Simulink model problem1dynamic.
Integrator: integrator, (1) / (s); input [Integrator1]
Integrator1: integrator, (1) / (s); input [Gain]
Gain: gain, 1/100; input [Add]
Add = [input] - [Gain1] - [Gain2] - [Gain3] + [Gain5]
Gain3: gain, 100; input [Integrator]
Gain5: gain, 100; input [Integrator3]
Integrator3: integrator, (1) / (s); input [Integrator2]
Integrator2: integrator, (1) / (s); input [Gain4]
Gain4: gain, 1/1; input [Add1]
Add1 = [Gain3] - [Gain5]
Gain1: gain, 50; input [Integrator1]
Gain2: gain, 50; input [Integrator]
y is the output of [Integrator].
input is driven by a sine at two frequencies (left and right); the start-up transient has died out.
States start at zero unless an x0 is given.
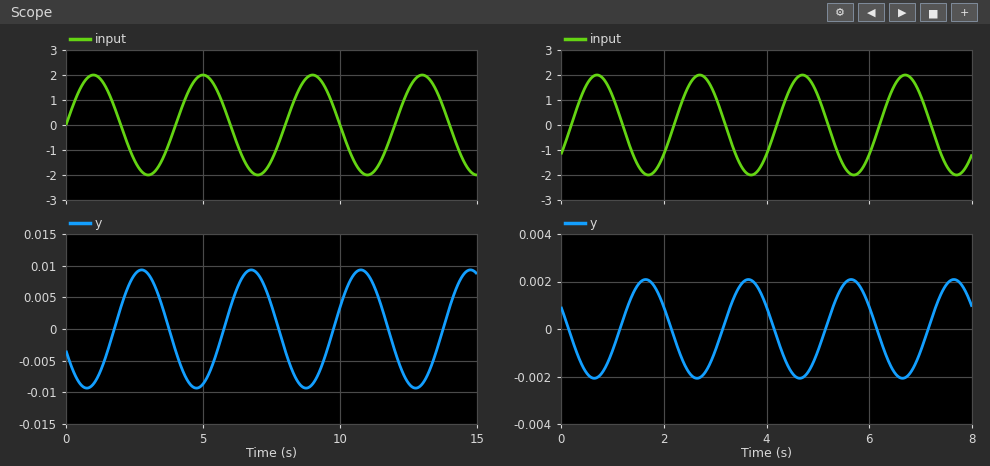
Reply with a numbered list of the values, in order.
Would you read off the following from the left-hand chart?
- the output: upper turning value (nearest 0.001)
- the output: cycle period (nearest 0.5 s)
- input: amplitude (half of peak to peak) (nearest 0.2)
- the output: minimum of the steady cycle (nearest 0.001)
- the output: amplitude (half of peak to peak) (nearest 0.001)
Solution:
1. 0.009
2. 4.0 s
3. 2.0
4. -0.009
5. 0.009
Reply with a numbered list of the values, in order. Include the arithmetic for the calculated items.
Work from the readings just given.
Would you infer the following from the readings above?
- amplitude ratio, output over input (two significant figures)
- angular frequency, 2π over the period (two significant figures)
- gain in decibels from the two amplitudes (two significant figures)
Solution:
1. 0.009 / 2 = 0.0045
2. 2π / 4 = 1.6 rad/s
3. 20 log10(0.009 / 2) = -47 dB
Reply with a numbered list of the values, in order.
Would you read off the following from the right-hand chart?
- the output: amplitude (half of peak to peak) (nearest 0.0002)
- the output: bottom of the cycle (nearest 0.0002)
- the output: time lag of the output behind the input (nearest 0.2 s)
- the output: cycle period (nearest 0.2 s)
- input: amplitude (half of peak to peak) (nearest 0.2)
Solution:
1. 0.0020
2. -0.0020
3. 1.0 s
4. 2.0 s
5. 2.0
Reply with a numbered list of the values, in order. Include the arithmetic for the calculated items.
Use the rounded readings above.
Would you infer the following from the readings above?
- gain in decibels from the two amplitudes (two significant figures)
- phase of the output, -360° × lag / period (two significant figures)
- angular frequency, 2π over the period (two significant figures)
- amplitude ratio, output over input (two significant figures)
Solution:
1. 20 log10(0.002 / 2) = -60 dB
2. -360 × 1 / 2 = -180°
3. 2π / 2 = 3.1 rad/s
4. 0.002 / 2 = 0.0010
